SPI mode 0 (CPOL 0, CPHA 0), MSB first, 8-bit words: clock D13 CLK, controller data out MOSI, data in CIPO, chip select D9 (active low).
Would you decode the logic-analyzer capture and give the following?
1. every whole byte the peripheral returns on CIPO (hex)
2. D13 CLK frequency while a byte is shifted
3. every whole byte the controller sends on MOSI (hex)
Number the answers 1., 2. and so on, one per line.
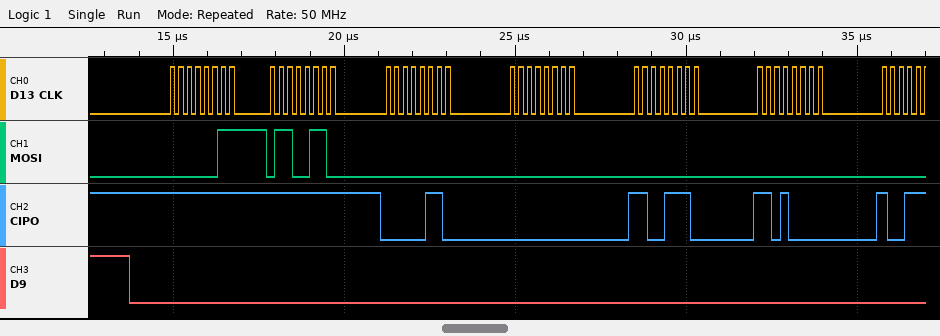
1. FF FF 06 00 CE D0
2. 4 MHz
3. 03 66 00 00 00 00
